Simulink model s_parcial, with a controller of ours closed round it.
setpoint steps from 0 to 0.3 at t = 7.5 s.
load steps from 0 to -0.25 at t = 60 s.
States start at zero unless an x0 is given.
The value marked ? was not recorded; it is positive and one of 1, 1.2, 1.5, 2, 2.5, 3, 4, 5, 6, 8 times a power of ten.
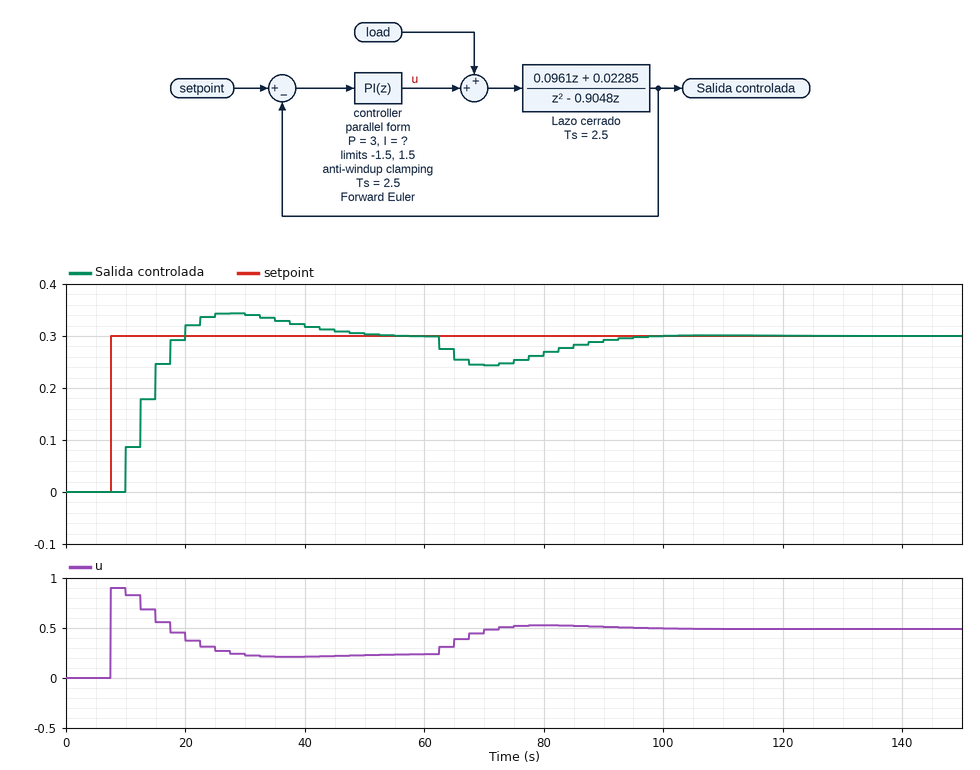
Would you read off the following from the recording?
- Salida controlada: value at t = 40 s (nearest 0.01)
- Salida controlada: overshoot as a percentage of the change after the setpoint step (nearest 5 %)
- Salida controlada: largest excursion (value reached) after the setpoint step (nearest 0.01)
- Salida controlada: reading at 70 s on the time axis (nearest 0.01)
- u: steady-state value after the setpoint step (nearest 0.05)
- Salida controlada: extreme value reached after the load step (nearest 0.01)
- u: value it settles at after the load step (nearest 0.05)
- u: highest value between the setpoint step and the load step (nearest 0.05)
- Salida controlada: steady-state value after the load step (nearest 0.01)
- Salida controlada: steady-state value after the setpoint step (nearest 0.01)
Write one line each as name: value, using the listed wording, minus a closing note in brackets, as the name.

Salida controlada: value at t = 40 s: 0.32
Salida controlada: overshoot as a percentage of the change after the setpoint step: 15 %
Salida controlada: largest excursion (value reached) after the setpoint step: 0.34
Salida controlada: reading at 70 s on the time axis: 0.24
u: steady-state value after the setpoint step: 0.25
Salida controlada: extreme value reached after the load step: 0.24
u: value it settles at after the load step: 0.50
u: highest value between the setpoint step and the load step: 0.90
Salida controlada: steady-state value after the load step: 0.30
Salida controlada: steady-state value after the setpoint step: 0.30
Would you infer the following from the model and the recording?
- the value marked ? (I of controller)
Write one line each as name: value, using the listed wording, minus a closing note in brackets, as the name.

the value marked ?: 0.25
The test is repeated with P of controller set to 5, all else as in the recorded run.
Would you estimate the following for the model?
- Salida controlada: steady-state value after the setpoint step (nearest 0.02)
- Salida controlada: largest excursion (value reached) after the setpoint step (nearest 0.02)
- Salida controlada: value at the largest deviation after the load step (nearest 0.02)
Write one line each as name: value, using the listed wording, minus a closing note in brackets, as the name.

Salida controlada: steady-state value after the setpoint step: 0.30
Salida controlada: largest excursion (value reached) after the setpoint step: 0.32
Salida controlada: value at the largest deviation after the load step: 0.26
